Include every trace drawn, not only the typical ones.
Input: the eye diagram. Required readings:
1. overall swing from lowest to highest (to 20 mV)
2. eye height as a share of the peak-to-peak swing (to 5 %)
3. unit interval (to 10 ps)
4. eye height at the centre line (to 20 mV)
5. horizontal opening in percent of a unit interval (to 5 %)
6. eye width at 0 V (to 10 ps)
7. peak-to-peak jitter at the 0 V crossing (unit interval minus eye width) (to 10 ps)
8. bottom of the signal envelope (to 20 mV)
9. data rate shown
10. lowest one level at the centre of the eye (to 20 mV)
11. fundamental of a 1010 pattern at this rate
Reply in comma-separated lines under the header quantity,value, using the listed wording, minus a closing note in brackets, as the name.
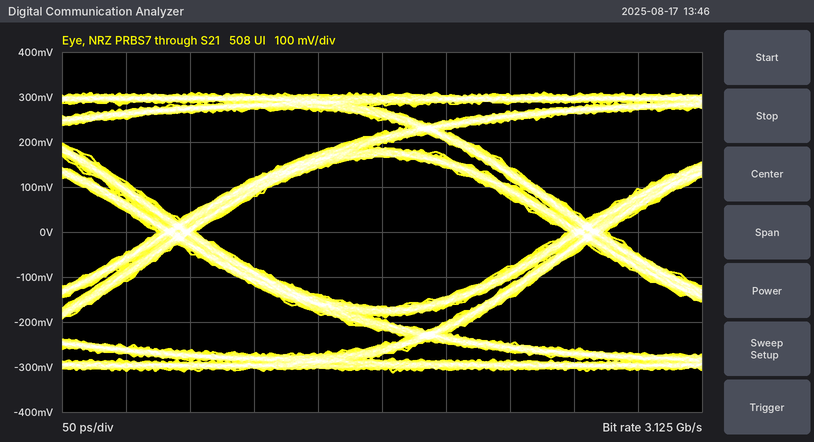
quantity,value
overall swing from lowest to highest,620 mV
eye height as a share of the peak-to-peak swing,55 %
unit interval,320 ps
eye height at the centre line,340 mV
horizontal opening in percent of a unit interval,90 %
eye width at 0 V,290 ps
peak-to-peak jitter at the 0 V crossing (unit interval minus eye width),30 ps
bottom of the signal envelope,-320 mV
data rate shown,3.125 Gb/s
lowest one level at the centre of the eye,160 mV
fundamental of a 1010 pattern at this rate,1.5625 GHz
